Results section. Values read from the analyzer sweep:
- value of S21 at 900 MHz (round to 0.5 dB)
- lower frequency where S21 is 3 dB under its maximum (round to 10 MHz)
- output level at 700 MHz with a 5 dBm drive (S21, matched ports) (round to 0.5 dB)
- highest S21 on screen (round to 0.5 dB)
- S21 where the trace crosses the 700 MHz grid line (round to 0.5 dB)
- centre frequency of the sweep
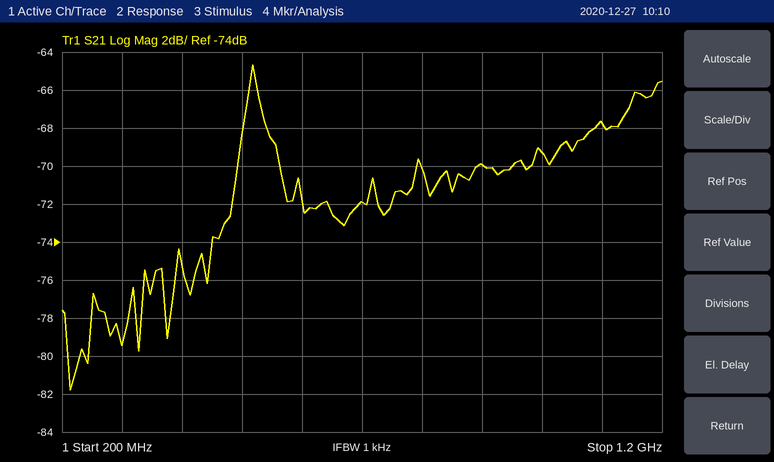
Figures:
-70.0 dB
500 MHz
-67.0 dBm
-64.5 dB
-72.0 dB
700 MHz
